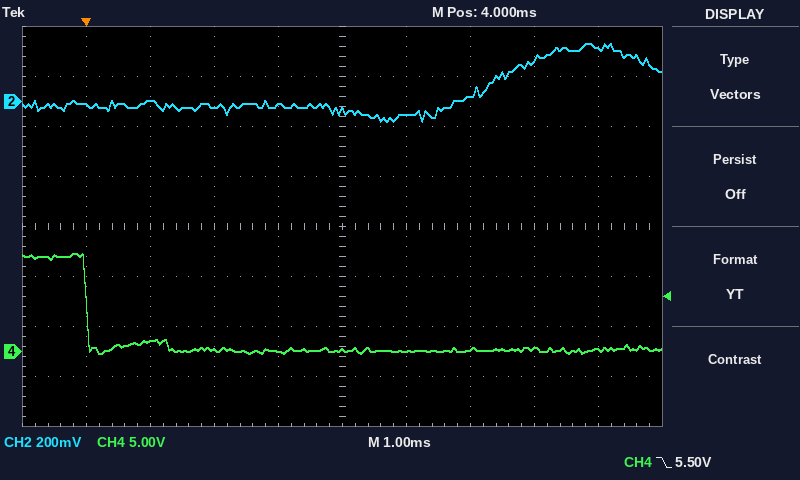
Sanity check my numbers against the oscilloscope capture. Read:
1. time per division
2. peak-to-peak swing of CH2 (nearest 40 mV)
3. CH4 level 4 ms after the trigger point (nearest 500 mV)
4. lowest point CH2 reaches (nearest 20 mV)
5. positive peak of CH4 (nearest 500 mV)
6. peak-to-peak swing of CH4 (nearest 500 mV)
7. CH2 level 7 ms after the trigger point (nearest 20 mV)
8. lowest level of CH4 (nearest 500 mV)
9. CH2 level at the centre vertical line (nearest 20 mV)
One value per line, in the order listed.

1 ms
320 mV
0.0 V
-80 mV
10.0 V
10.0 V
160 mV
0.0 V
-40 mV
